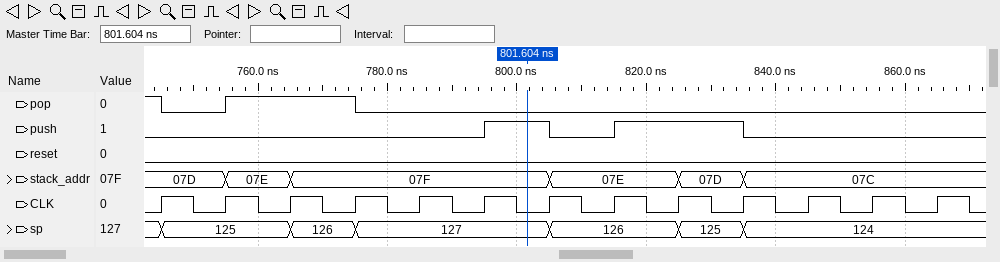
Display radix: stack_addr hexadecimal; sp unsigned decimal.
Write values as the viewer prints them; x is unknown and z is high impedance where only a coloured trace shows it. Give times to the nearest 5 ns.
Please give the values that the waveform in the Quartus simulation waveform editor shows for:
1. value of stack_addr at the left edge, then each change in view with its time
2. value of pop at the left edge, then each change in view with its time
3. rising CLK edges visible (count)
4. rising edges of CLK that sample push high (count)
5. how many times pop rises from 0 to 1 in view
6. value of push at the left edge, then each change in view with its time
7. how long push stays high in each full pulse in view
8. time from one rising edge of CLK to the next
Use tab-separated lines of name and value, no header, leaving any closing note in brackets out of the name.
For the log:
value of stack_addr at the left edge, then each change in view with its time	07D, 07E at 755 ns, 07F at 765 ns, 07E at 805 ns, 07D at 825 ns, 07C at 835 ns
value of pop at the left edge, then each change in view with its time	1, 0 at 745 ns, 1 at 755 ns, 0 at 775 ns
rising CLK edges visible	13
rising edges of CLK that sample push high	3
how many times pop rises from 0 to 1 in view	1
value of push at the left edge, then each change in view with its time	0, 1 at 795 ns, 0 at 805 ns, 1 at 815 ns, 0 at 835 ns
how long push stays high in each full pulse in view	10 ns, 20 ns
time from one rising edge of CLK to the next	10 ns
